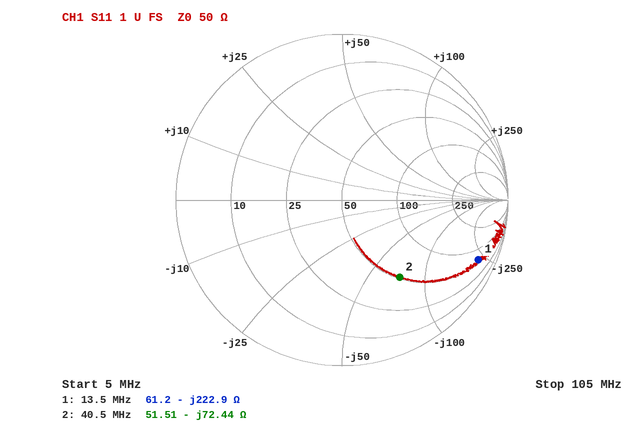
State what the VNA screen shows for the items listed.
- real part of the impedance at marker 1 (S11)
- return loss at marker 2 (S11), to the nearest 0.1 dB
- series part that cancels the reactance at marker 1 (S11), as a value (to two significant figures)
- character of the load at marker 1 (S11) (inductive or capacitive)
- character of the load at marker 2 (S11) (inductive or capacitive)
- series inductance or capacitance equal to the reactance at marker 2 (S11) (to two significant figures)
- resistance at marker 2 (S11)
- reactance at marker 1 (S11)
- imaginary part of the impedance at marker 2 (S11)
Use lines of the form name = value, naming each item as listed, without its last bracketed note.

real part of the impedance at marker 1 = 61.2 Ω
return loss at marker 2 (S11), to the nearest 0.1 dB = 4.7 dB
series part that cancels the reactance at marker 1 (S11), as a value = 2.6 µH
character of the load at marker 1 (S11) = capacitive
character of the load at marker 2 (S11) = capacitive
series inductance or capacitance equal to the reactance at marker 2 (S11) = 54 pF
resistance at marker 2 = 51.51 Ω
reactance at marker 1 = -222.9 Ω
imaginary part of the impedance at marker 2 = -72.44 Ω
